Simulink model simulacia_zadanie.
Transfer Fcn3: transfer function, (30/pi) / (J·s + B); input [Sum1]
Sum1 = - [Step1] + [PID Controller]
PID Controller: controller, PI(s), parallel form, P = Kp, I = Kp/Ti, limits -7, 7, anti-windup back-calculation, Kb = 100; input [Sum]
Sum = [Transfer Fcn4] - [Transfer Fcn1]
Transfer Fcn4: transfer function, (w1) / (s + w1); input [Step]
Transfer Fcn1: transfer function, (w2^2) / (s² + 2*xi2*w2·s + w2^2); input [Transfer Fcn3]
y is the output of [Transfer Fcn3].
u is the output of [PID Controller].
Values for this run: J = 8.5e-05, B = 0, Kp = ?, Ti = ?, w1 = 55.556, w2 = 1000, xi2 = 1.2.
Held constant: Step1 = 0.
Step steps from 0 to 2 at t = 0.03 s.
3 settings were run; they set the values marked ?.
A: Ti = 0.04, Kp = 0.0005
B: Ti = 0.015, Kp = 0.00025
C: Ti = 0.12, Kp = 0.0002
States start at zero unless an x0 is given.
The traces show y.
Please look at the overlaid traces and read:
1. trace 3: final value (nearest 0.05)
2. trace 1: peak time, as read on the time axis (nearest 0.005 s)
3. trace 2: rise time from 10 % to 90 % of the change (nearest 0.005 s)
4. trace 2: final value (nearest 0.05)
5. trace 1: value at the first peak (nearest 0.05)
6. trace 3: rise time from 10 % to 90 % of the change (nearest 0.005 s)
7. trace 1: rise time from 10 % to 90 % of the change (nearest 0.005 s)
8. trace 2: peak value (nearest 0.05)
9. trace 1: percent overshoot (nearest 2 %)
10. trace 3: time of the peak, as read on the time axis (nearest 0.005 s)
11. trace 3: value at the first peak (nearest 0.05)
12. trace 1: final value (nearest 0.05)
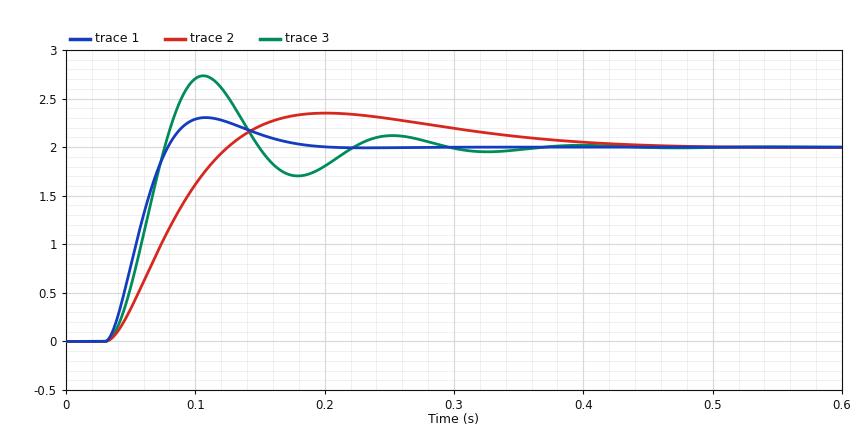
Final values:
2.00
0.110 s
0.065 s
2.00
2.30
0.030 s
0.035 s
2.35
16 %
0.105 s
2.75
2.00
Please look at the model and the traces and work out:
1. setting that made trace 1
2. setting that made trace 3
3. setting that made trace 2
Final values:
A
B
C
